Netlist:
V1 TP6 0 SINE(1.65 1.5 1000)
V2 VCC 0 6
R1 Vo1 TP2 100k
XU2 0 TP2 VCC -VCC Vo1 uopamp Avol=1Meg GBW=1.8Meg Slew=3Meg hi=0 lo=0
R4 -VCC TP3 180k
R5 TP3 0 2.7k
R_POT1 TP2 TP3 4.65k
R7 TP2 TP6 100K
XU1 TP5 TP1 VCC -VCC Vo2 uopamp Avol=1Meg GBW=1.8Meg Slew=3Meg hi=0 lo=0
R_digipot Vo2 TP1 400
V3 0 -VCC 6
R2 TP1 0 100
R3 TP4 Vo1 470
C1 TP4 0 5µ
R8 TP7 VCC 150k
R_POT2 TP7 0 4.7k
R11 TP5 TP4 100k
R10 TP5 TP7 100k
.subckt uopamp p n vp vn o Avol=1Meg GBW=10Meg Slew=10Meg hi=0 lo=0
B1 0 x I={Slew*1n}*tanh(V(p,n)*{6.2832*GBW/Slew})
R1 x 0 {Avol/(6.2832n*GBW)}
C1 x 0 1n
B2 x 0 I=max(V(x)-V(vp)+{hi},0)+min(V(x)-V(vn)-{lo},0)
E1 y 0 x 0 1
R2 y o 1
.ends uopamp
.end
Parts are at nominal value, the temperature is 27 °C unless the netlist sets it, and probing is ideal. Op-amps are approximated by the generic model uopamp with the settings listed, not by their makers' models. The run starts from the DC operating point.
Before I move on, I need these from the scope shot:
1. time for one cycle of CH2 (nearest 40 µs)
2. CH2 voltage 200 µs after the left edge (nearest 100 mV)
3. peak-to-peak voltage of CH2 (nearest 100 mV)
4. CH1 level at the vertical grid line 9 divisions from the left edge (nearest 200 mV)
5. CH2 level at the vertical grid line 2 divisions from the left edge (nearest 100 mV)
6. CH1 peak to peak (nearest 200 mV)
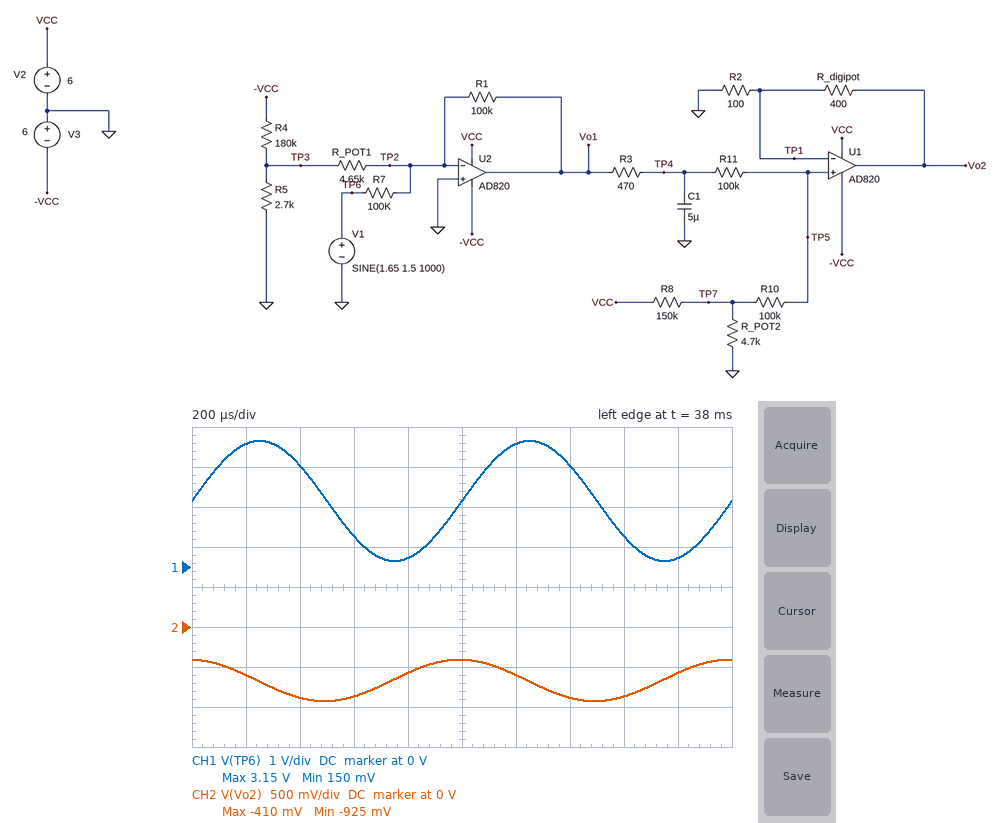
1.00 ms
-600 mV
500 mV
200 mV
-900 mV
3.0 V
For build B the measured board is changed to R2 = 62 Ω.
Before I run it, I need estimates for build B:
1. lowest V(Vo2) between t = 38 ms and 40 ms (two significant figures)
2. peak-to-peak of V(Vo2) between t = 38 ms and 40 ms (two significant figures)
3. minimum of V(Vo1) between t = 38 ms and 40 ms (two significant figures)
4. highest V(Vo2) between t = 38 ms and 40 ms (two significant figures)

-1.4 V
770 mV
-1.9 V
-610 mV
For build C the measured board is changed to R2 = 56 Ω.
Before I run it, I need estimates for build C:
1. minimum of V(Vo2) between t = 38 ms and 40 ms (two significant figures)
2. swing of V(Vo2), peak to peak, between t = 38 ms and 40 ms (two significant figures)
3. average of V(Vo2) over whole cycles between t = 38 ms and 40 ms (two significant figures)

-1.5 V
840 mV
-1.1 V
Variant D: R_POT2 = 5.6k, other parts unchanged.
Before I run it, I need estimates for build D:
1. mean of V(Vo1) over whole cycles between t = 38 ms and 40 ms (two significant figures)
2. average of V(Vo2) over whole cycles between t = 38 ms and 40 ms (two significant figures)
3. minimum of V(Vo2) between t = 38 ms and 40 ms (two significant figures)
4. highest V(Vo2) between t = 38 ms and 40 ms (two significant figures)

-440 mV
-590 mV
-850 mV
-330 mV
